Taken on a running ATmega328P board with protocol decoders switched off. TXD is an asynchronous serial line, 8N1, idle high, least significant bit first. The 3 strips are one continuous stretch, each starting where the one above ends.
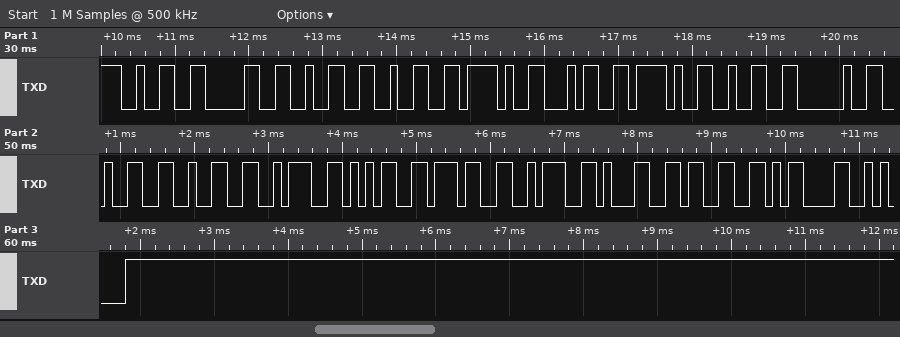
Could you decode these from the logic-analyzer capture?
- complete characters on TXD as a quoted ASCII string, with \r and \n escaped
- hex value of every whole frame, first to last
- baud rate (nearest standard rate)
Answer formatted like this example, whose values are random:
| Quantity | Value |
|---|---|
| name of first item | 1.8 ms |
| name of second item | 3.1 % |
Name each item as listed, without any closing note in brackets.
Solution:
| Quantity | Value |
|---|---|
| complete characters on TXD as a quoted ASCII string, with \r and \n escaped | "2022/4/2 22:57:13\r\n" |
| hex value of every whole frame, first to last | 32 30 32 32 2F 34 2F 32 20 32 32 3A 35 37 3A 31 33 0D 0A |
| baud rate | 9600 baud |
